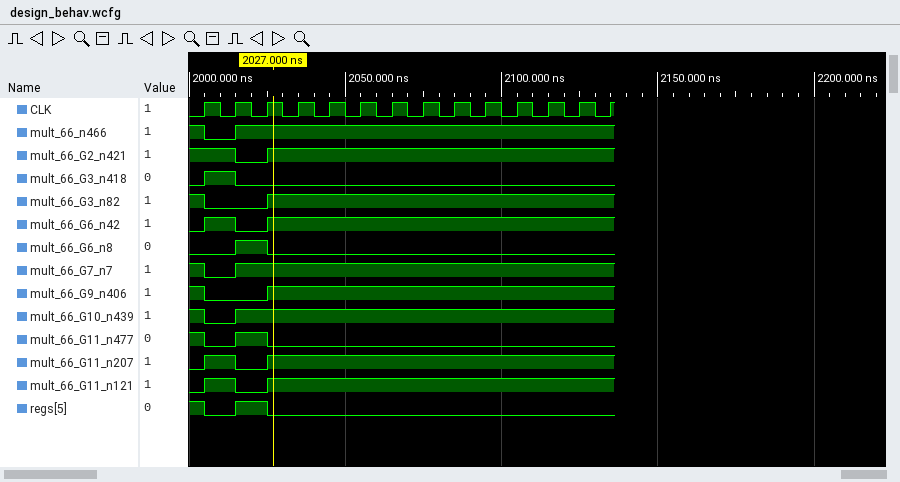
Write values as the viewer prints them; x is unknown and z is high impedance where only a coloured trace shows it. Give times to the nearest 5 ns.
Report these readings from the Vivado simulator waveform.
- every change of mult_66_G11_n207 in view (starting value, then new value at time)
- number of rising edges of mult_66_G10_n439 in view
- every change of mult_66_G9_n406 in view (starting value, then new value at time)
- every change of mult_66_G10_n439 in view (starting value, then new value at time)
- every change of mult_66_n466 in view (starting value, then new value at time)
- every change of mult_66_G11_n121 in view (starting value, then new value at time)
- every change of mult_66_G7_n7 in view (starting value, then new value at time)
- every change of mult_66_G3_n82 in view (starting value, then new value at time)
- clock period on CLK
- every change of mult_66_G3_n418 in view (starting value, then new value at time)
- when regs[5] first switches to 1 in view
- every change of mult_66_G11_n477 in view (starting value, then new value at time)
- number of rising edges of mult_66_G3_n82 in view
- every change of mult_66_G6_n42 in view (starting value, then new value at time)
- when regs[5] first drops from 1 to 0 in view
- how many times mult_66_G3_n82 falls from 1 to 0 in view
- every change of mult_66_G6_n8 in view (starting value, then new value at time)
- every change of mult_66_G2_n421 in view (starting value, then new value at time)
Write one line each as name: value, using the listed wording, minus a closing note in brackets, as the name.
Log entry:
every change of mult_66_G11_n207 in view: 0, 1 at 2005 ns, 0 at 2015 ns, 1 at 2025 ns
number of rising edges of mult_66_G10_n439 in view: 1
every change of mult_66_G9_n406 in view: 1, 0 at 2005 ns, 1 at 2025 ns
every change of mult_66_G10_n439 in view: 1, 0 at 2005 ns, 1 at 2015 ns
every change of mult_66_n466 in view: 1, 0 at 2005 ns, 1 at 2015 ns
every change of mult_66_G11_n121 in view: 0, 1 at 2005 ns, 0 at 2015 ns, 1 at 2025 ns
every change of mult_66_G7_n7 in view: 1, 0 at 2005 ns, 1 at 2015 ns
every change of mult_66_G3_n82 in view: 1, 0 at 2005 ns, 1 at 2025 ns
clock period on CLK: 10 ns
every change of mult_66_G3_n418 in view: 0, 1 at 2005 ns, 0 at 2015 ns
when regs[5] first switches to 1 in view: 2015 ns
every change of mult_66_G11_n477 in view: 1, 0 at 2005 ns, 1 at 2015 ns, 0 at 2025 ns
number of rising edges of mult_66_G3_n82 in view: 1
every change of mult_66_G6_n42 in view: 0, 1 at 2005 ns, 0 at 2015 ns, 1 at 2025 ns
when regs[5] first drops from 1 to 0 in view: 2005 ns
how many times mult_66_G3_n82 falls from 1 to 0 in view: 1
every change of mult_66_G6_n8 in view: 0, 1 at 2015 ns, 0 at 2025 ns
every change of mult_66_G2_n421 in view: 1, 0 at 2015 ns, 1 at 2025 ns
